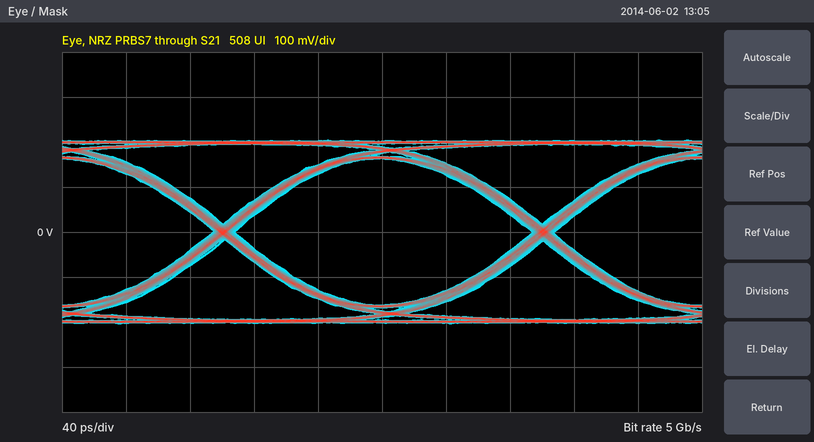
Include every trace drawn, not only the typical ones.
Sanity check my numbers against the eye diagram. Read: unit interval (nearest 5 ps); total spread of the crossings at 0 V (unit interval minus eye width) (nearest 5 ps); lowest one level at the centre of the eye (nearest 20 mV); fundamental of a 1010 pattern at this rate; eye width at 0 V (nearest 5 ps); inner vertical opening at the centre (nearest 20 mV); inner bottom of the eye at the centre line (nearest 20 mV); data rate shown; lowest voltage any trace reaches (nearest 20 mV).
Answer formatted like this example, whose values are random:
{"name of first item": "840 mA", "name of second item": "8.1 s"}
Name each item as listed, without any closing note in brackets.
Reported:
{"unit interval": "200 ps", "total spread of the crossings at 0 V (unit interval minus eye width)": "15 ps", "lowest one level at the centre of the eye": "160 mV", "fundamental of a 1010 pattern at this rate": "2.5 GHz", "eye width at 0 V": "185 ps", "inner vertical opening at the centre": "320 mV", "inner bottom of the eye at the centre line": "-160 mV", "data rate shown": "5 Gb/s", "lowest voltage any trace reaches": "-200 mV"}
